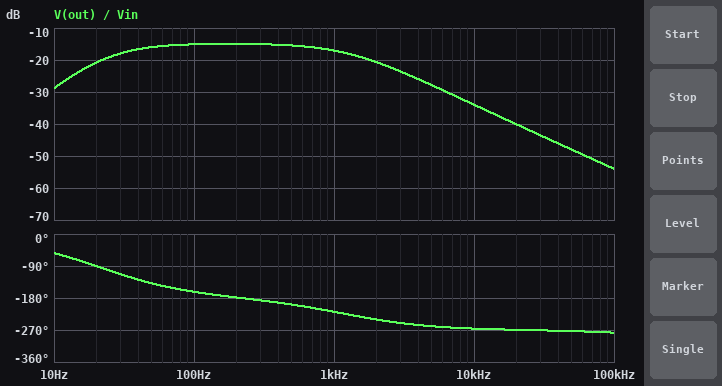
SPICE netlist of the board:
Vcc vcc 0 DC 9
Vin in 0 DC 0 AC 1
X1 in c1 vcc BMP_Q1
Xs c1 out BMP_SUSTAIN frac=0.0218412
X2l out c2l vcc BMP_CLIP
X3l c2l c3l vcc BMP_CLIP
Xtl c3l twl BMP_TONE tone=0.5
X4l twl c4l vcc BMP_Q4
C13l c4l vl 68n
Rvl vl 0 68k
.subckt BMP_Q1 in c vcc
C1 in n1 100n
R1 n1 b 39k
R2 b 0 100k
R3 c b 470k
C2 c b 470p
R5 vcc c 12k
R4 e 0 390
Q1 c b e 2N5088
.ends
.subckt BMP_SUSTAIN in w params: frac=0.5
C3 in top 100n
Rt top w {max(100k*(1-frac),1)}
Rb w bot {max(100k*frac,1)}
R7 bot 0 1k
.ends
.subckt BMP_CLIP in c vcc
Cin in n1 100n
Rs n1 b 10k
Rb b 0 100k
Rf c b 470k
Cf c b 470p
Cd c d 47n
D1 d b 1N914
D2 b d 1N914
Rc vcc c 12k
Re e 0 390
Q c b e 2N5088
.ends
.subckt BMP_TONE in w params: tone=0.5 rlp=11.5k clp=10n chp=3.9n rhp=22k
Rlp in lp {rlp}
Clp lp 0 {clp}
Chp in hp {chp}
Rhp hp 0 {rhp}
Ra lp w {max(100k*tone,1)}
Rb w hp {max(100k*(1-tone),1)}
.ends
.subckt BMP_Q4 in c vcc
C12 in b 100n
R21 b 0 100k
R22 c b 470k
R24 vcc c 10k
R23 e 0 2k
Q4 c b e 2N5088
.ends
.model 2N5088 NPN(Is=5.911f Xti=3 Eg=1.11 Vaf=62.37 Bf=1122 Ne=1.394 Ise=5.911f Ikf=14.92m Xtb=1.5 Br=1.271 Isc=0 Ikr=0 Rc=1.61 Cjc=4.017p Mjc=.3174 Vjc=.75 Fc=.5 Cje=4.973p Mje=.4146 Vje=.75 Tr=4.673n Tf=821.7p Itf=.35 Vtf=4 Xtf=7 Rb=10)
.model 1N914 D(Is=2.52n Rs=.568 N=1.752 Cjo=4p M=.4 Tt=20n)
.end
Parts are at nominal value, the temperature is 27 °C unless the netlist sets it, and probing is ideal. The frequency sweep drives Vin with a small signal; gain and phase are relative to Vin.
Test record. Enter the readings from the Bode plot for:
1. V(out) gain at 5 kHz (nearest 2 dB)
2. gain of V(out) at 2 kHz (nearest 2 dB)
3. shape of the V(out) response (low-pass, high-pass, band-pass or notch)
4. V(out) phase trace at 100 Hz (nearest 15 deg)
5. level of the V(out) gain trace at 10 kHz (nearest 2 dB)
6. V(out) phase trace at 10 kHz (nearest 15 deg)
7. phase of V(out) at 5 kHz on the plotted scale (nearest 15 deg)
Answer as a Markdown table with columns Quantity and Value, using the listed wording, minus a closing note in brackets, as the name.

| Quantity | Value |
|---|---|
| V(out) gain at 5 kHz | -28 dB |
| gain of V(out) at 2 kHz | -20 dB |
| shape of the V(out) response | band-pass |
| V(out) phase trace at 100 Hz | -165 deg |
| level of the V(out) gain trace at 10 kHz | -34 dB |
| V(out) phase trace at 10 kHz | -270 deg |
| phase of V(out) at 5 kHz on the plotted scale | -255 deg |
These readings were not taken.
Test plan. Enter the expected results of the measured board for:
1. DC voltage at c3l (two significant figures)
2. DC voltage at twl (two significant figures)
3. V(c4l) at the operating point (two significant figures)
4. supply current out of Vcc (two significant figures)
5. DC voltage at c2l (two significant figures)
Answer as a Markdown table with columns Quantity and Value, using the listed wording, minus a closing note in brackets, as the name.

| Quantity | Value |
|---|---|
| DC voltage at c3l | 4.6 V |
| DC voltage at twl | 2.5 V |
| V(c4l) at the operating point | 6.5 V |
| supply current out of Vcc | 1.3 mA |
| DC voltage at c2l | 4.7 V |
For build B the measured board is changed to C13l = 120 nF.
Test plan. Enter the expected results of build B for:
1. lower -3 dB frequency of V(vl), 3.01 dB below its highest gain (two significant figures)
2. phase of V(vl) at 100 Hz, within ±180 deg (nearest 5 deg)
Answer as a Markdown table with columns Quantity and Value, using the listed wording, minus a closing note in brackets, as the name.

| Quantity | Value |
|---|---|
| lower -3 dB frequency of V(vl), 3.01 dB below its highest gain | 76 Hz |
| phase of V(vl) at 100 Hz, within ±180 deg | 85 deg |
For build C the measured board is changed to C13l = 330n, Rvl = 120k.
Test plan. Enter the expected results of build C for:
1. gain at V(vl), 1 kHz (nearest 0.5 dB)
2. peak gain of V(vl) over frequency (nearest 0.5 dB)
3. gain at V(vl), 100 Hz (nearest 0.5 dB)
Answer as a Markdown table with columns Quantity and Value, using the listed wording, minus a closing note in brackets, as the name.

| Quantity | Value |
|---|---|
| gain at V(vl), 1 kHz | 23.0 dB |
| peak gain of V(vl) over frequency | 29.5 dB |
| gain at V(vl), 100 Hz | 28.0 dB |
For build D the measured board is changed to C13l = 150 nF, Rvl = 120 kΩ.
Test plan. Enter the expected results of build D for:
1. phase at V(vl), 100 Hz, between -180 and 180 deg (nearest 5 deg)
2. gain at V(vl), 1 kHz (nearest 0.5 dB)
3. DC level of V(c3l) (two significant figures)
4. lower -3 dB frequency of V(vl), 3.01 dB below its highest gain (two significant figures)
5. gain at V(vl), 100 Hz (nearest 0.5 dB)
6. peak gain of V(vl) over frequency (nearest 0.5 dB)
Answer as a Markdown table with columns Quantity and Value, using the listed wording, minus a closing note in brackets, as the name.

| Quantity | Value |
|---|---|
| phase at V(vl), 100 Hz, between -180 and 180 deg | 80 deg |
| gain at V(vl), 1 kHz | 23.0 dB |
| DC level of V(c3l) | 4.6 V |
| lower -3 dB frequency of V(vl), 3.01 dB below its highest gain | 75 Hz |
| gain at V(vl), 100 Hz | 28.0 dB |
| peak gain of V(vl) over frequency | 29.5 dB |
